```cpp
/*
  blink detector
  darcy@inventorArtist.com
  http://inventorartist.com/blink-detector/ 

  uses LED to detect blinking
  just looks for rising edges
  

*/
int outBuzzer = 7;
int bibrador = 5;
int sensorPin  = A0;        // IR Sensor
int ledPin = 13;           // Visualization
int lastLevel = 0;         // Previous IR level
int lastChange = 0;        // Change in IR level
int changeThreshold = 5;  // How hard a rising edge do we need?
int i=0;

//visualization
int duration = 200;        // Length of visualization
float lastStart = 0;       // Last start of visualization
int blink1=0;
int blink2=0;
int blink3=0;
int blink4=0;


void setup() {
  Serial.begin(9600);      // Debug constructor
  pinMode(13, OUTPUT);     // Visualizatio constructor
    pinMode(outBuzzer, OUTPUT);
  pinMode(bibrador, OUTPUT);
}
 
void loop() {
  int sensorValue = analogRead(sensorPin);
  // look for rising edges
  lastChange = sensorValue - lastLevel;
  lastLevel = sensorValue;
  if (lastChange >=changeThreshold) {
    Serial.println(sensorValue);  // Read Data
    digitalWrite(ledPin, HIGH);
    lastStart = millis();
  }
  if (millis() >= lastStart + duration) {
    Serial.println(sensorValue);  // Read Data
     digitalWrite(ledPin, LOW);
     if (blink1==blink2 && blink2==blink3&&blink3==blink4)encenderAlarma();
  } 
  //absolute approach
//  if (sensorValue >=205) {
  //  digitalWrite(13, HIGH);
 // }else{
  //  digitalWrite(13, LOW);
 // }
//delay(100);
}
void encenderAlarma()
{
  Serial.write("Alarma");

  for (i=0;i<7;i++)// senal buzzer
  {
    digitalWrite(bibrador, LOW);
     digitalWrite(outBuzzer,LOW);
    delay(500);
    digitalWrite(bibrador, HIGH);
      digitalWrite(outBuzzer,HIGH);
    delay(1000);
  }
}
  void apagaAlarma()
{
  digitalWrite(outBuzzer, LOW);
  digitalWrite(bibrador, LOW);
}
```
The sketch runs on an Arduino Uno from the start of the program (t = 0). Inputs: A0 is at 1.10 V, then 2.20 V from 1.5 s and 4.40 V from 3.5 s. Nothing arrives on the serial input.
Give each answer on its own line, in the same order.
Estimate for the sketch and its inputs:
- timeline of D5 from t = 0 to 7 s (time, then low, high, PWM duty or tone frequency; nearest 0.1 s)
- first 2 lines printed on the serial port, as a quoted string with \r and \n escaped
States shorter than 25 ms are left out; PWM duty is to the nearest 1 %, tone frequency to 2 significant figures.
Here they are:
0 s low; 0.7 s high; 1.7 s low; 2.2 s high; 3.2 s low; 3.7 s high; 4.7 s low; 5.2 s high; 6.2 s low; 6.7 s high
"225\r\n225\r\n"
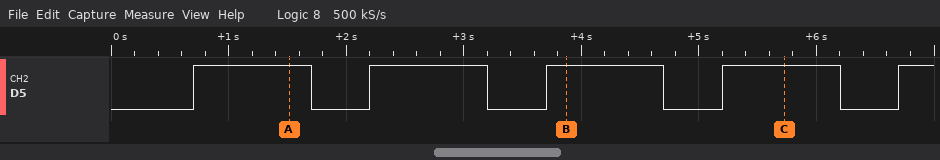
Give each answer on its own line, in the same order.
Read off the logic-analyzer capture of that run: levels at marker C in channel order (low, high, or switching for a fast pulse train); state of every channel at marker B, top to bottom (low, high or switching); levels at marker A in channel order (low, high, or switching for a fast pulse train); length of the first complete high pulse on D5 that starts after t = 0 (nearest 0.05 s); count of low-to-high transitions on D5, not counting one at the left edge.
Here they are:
D5 high
D5 high
D5 high
1.00 s
5
